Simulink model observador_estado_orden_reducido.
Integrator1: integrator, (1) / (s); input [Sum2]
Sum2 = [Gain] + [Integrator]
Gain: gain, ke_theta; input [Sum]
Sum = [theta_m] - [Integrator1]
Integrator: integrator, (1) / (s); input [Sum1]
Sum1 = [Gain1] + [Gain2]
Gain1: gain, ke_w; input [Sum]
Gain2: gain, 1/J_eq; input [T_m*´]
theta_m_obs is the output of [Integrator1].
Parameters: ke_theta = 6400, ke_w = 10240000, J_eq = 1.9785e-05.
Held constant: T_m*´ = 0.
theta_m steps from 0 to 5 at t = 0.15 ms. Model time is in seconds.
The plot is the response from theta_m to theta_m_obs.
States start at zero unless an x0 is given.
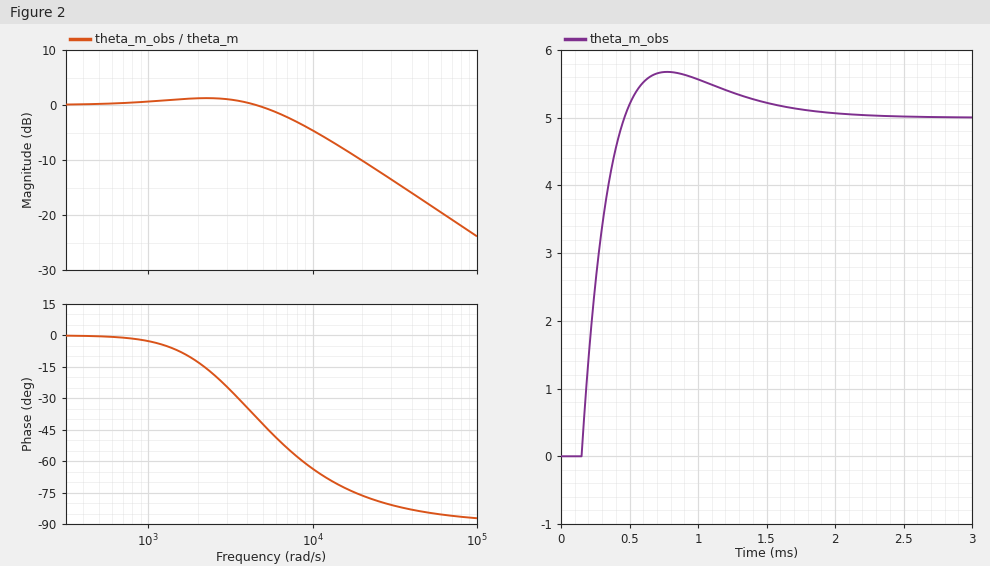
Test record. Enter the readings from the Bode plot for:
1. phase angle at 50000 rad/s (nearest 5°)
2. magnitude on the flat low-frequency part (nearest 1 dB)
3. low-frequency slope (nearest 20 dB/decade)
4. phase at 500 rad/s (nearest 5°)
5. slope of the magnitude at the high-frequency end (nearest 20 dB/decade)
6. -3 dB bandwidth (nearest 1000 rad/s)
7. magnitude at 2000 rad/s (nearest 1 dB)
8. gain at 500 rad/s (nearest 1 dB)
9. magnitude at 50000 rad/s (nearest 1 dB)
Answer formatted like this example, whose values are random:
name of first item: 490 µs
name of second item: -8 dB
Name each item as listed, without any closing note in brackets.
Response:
phase angle at 50000 rad/s: -85°
magnitude on the flat low-frequency part: 0 dB
low-frequency slope: 0 dB/decade
phase at 500 rad/s: 0°
slope of the magnitude at the high-frequency end: -20 dB/decade
-3 dB bandwidth: 8000 rad/s
magnitude at 2000 rad/s: 1 dB
gain at 500 rad/s: 0 dB
magnitude at 50000 rad/s: -18 dB
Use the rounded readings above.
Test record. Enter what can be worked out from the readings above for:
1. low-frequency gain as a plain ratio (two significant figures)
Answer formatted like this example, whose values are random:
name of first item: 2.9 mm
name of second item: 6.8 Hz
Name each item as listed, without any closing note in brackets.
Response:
low-frequency gain as a plain ratio: 1.0
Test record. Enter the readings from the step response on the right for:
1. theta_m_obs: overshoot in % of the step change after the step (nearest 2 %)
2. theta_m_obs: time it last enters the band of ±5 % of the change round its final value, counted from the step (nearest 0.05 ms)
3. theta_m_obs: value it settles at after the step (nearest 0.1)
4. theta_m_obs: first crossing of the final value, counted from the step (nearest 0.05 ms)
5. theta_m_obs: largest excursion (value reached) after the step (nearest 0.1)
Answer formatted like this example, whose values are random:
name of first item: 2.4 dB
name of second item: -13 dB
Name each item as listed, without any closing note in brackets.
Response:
theta_m_obs: overshoot in % of the step change after the step: 14 %
theta_m_obs: time it last enters the band of ±5 % of the change round its final value, counted from the step: 1.30 ms
theta_m_obs: value it settles at after the step: 5.0
theta_m_obs: first crossing of the final value, counted from the step: 0.30 ms
theta_m_obs: largest excursion (value reached) after the step: 5.7
